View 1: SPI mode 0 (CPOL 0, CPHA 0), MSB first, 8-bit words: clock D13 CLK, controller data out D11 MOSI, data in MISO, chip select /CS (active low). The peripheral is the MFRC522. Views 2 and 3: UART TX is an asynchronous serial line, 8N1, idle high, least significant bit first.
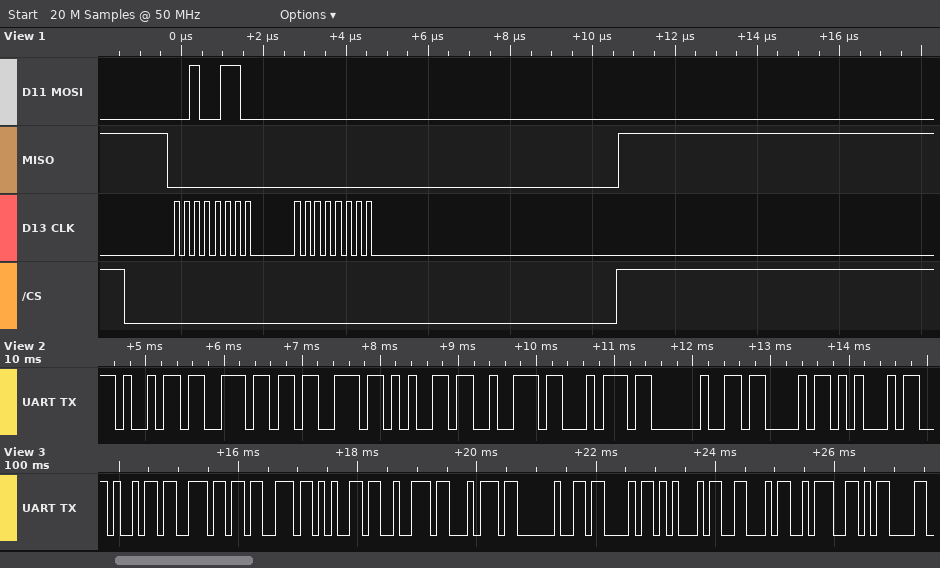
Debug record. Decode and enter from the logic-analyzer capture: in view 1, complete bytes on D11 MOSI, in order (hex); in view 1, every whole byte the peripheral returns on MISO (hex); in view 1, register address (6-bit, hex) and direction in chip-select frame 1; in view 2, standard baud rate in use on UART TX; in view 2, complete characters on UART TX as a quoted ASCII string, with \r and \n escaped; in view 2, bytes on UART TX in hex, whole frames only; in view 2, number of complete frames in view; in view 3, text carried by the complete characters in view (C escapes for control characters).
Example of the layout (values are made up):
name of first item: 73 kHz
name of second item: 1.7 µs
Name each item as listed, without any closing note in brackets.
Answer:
in view 1, complete bytes on D11 MOSI, in order: 26 00
in view 1, every whole byte the peripheral returns on MISO: 00 00
in view 1, register address (6-bit, hex) and direction in chip-select frame 1: 0x13 write
in view 2, standard baud rate in use on UART TX: 9600 baud
in view 2, complete characters on UART TX as a quoted ASCII string, with \r and \n escaped: "insert CE"
in view 2, bytes on UART TX in hex, whole frames only: 69 6E 73 65 72 74 20 43 45
in view 2, number of complete frames in view: 9
in view 3, text carried by the complete characters in view: "insert CEF:\r"
